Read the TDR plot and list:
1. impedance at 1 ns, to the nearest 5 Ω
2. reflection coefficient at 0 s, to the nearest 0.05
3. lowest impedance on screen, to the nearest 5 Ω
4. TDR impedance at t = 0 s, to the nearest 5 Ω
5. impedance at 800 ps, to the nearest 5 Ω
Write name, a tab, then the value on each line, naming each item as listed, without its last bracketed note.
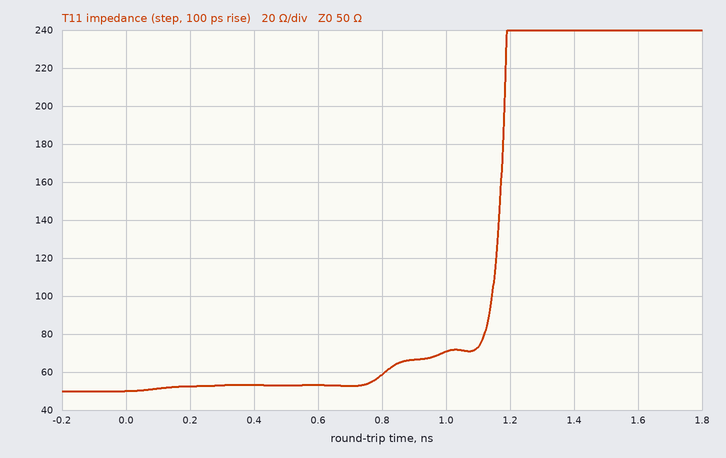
impedance at 1 ns, to the nearest 5 Ω	70 Ω
reflection coefficient at 0 s, to the nearest 0.05	0.00
lowest impedance on screen, to the nearest 5 Ω	50 Ω
TDR impedance at t = 0 s, to the nearest 5 Ω	50 Ω
impedance at 800 ps, to the nearest 5 Ω	60 Ω
